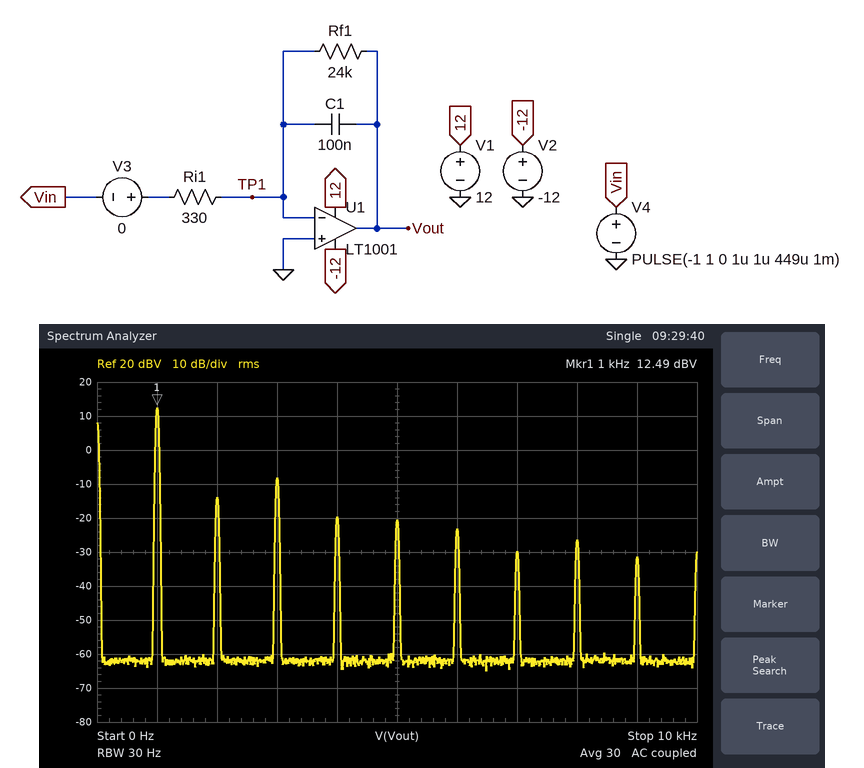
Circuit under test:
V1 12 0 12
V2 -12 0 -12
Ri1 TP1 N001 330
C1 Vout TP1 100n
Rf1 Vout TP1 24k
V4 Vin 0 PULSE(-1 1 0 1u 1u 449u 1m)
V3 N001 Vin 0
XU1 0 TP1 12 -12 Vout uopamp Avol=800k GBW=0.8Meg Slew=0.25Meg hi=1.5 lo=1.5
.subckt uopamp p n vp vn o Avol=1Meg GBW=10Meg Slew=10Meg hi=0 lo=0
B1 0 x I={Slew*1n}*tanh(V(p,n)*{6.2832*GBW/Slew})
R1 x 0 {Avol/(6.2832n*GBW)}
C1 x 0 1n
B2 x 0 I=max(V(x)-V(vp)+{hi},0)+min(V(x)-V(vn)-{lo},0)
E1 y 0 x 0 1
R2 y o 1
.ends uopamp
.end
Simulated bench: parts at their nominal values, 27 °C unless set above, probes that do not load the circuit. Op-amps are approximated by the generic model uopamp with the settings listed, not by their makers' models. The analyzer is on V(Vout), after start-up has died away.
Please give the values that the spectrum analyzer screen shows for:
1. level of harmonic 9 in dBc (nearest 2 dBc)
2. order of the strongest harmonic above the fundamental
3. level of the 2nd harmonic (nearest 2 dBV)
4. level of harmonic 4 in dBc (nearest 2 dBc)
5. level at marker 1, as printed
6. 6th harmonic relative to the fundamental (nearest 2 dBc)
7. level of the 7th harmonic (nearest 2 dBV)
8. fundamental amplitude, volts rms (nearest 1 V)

-44 dBc
3
-14 dBV
-32 dBc
12.49 dBV
-36 dBc
-30 dBV
4 V
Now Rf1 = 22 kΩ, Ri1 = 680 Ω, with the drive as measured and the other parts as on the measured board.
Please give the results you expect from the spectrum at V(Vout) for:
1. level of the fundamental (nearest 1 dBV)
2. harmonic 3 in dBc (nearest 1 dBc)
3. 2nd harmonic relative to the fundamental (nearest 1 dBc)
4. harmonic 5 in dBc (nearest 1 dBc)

6 dBV
-20 dBc
-22 dBc
-31 dBc
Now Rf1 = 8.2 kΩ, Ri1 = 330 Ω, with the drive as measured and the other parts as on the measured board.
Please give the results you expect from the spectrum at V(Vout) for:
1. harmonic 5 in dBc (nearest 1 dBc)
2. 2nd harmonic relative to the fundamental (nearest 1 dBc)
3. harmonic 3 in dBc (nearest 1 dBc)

-31 dBc
-22 dBc
-20 dBc
